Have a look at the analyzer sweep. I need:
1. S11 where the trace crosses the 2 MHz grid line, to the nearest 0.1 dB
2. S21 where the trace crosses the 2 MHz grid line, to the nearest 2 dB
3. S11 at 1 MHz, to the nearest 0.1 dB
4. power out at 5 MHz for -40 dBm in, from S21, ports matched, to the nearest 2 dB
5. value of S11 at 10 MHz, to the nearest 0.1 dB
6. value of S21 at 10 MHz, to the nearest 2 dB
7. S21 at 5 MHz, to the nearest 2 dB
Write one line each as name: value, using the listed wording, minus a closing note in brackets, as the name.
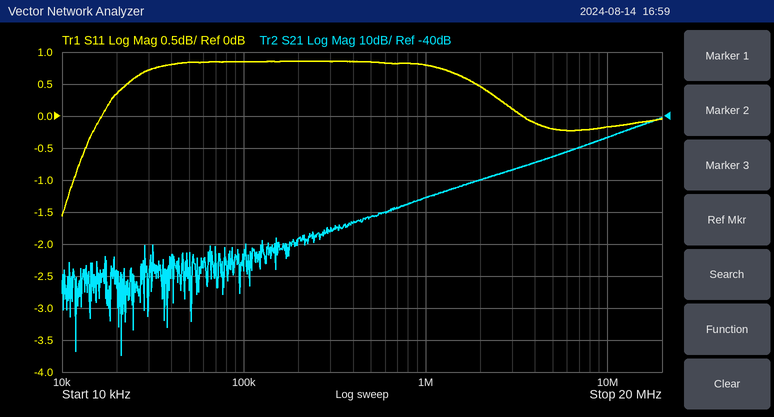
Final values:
S11 where the trace crosses the 2 MHz grid line, to the nearest 0.1 dB: 0.5 dB
S21 where the trace crosses the 2 MHz grid line, to the nearest 2 dB: -60 dB
S11 at 1 MHz, to the nearest 0.1 dB: 0.8 dB
power out at 5 MHz for -40 dBm in, from S21, ports matched, to the nearest 2 dB: -92 dBm
value of S11 at 10 MHz, to the nearest 0.1 dB: -0.2 dB
value of S21 at 10 MHz, to the nearest 2 dB: -46 dB
S21 at 5 MHz, to the nearest 2 dB: -52 dB
